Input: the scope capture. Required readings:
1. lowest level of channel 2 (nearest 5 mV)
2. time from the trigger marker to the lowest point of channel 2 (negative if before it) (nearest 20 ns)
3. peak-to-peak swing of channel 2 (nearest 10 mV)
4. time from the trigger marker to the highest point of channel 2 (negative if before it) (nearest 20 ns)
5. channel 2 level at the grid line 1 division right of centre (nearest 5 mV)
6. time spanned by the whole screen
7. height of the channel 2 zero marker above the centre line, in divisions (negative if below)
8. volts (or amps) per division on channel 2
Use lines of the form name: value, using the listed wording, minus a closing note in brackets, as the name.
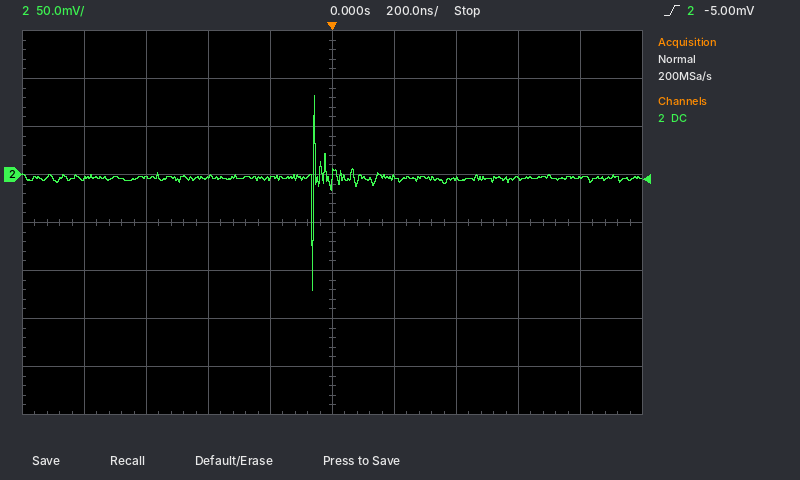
lowest level of channel 2: -120 mV
time from the trigger marker to the lowest point of channel 2 (negative if before it): -60 ns
peak-to-peak swing of channel 2: 200 mV
time from the trigger marker to the highest point of channel 2 (negative if before it): -60 ns
channel 2 level at the grid line 1 division right of centre: -5 mV
time spanned by the whole screen: 2 µs
height of the channel 2 zero marker above the centre line, in divisions: +1.0 div
volts (or amps) per division on channel 2: 50 mV
